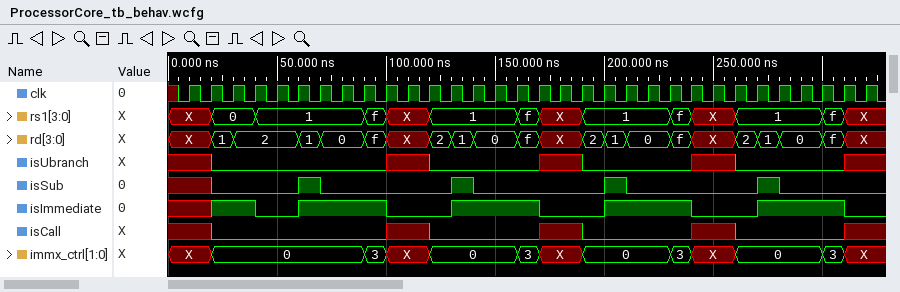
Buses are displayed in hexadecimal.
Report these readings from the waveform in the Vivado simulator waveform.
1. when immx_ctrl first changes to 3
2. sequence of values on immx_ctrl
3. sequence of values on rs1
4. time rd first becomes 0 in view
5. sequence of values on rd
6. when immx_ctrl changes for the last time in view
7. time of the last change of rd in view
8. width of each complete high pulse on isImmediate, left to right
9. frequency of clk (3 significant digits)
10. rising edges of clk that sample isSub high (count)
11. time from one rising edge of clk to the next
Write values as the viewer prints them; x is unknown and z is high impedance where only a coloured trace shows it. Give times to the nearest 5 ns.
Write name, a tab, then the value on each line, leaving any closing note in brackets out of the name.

when immx_ctrl first changes to 3	90 ns
sequence of values on immx_ctrl	X, 0, 3, X, 0, 3, X, 0, 3, X, 0, 3, X
sequence of values on rs1	X, 0, 1, f, X, 1, f, X, 1, f, X, 1, f, X
time rd first becomes 0 in view	70 ns
sequence of values on rd	X, 1, 2, 1, 0, f, X, 2, 1, 0, f, X, 2, 1, 0, f, X, 2, 1, 0, f, X
when immx_ctrl changes for the last time in view	310 ns
time of the last change of rd in view	310 ns
width of each complete high pulse on isImmediate, left to right	40 ns, 40 ns, 40 ns, 40 ns
frequency of clk	100 MHz
rising edges of clk that sample isSub high	4
time from one rising edge of clk to the next	10 ns
